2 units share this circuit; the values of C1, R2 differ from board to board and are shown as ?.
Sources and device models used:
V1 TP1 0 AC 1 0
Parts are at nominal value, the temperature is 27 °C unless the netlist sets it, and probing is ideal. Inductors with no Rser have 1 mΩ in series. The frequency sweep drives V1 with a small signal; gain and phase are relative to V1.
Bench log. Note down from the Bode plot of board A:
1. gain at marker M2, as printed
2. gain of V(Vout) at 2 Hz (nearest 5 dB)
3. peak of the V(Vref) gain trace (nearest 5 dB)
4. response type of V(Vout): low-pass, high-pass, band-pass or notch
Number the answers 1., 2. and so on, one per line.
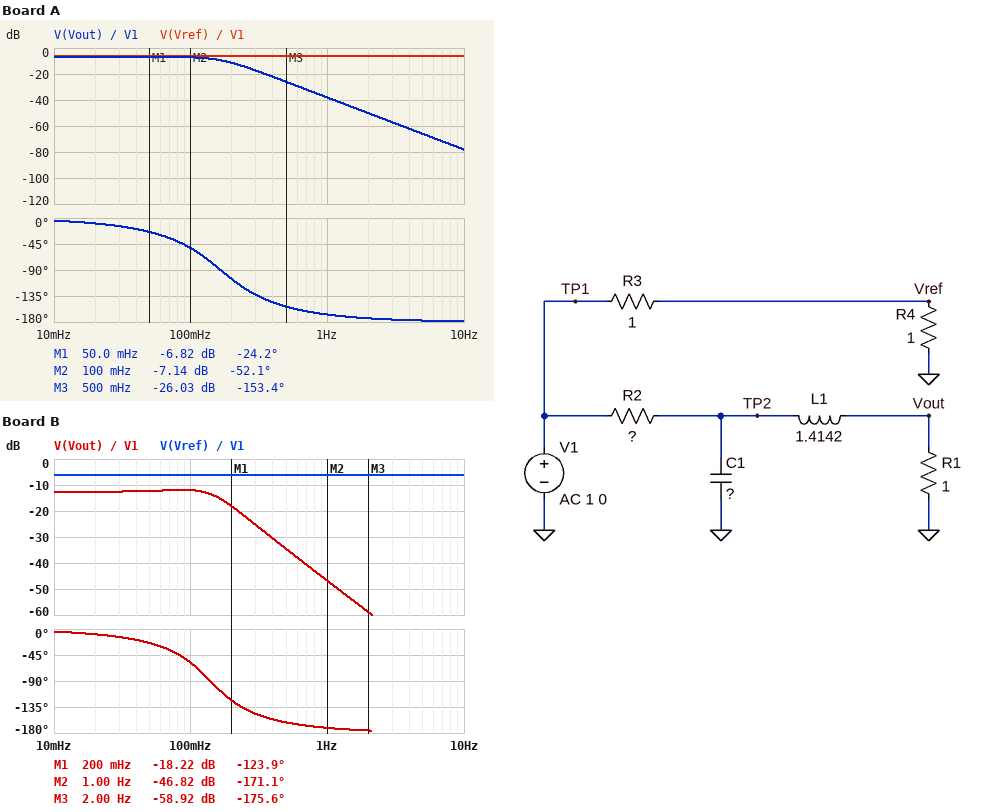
1. -7.14 dB
2. -50 dB
3. -5 dB
4. low-pass
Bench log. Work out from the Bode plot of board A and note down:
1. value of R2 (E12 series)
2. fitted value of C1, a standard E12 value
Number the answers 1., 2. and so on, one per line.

1. 1.2 Ω
2. 1.2 F
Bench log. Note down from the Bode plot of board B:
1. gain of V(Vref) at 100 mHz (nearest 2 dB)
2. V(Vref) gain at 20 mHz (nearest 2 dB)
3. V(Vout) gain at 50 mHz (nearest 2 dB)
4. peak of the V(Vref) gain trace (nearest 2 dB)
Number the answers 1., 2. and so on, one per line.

1. -6 dB
2. -6 dB
3. -12 dB
4. -6 dB
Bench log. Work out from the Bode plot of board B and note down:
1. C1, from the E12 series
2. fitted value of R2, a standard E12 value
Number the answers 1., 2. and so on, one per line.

1. 1.2 F
2. 3.3 Ω
